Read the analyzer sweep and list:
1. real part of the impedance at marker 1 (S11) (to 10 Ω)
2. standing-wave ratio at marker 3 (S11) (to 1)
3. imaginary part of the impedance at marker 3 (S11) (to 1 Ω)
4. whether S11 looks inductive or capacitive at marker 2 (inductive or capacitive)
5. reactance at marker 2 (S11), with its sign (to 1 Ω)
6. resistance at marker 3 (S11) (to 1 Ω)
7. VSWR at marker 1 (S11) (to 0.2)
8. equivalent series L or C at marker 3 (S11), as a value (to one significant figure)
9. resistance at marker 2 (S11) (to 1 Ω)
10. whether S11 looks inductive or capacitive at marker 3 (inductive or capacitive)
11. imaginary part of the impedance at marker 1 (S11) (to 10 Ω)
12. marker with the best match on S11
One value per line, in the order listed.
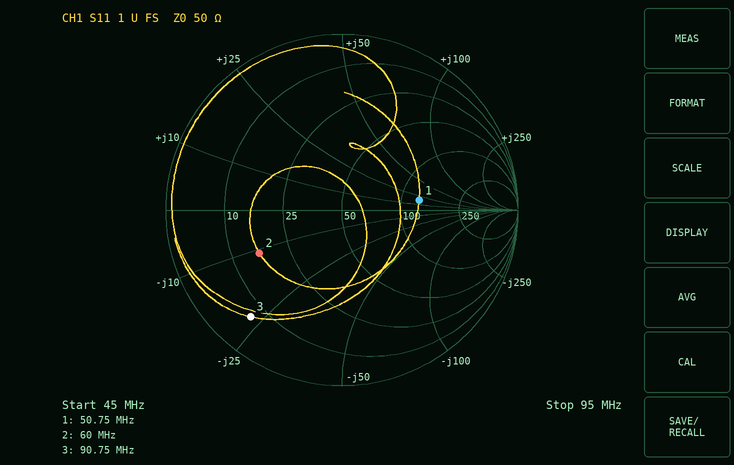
130 Ω
9
-23 Ω
capacitive
-11 Ω
7 Ω
2.6
80 pF
16 Ω
capacitive
+20 Ω
marker 1
